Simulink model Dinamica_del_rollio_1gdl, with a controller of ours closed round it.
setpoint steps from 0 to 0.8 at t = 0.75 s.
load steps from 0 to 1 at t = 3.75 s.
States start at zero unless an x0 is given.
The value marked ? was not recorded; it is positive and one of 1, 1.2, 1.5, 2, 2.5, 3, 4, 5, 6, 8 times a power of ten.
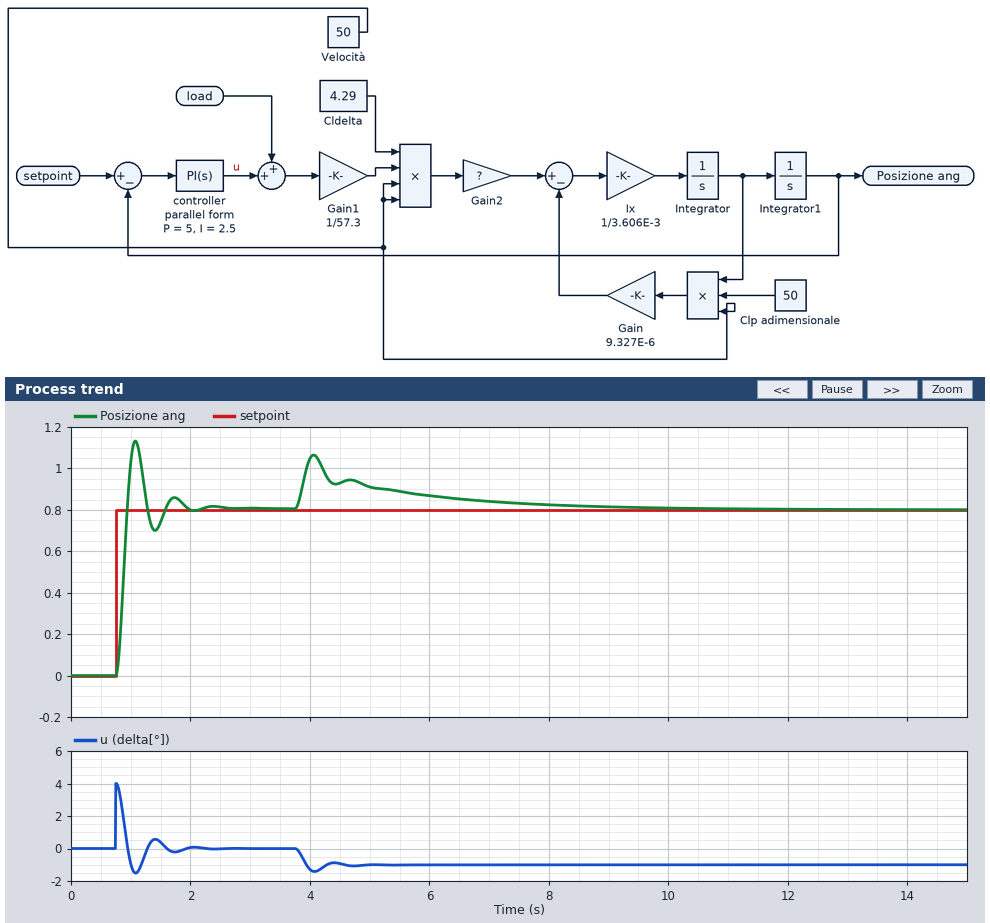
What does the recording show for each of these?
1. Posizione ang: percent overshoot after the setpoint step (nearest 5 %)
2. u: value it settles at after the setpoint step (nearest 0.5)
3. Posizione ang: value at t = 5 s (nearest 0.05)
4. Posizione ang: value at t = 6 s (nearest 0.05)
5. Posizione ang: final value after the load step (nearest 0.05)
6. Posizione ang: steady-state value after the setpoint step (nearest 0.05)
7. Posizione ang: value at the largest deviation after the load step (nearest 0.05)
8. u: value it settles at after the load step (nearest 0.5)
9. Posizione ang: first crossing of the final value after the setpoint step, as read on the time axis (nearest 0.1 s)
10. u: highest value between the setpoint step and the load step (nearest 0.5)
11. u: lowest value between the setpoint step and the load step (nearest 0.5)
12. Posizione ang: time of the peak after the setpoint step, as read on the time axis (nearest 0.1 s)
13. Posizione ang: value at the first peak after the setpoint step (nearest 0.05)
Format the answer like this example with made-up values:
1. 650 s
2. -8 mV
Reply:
1. 40 %
2. 0.0
3. 0.90
4. 0.85
5. 0.80
6. 0.80
7. 1.05
8. -1.0
9. 0.9 s
10. 4.0
11. -1.5
12. 1.1 s
13. 1.15
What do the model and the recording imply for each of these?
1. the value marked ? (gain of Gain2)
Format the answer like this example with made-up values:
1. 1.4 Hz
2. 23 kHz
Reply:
1. 0.0004
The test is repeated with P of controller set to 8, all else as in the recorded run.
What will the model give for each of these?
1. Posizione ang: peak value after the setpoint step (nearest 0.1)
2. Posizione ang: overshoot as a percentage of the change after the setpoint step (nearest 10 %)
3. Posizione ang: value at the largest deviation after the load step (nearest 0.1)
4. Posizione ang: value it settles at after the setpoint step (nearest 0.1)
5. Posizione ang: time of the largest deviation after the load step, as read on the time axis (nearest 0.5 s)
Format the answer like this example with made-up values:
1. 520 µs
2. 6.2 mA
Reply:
1. 1.2
2. 50 %
3. 1.0
4. 0.8
5. 4.0 s
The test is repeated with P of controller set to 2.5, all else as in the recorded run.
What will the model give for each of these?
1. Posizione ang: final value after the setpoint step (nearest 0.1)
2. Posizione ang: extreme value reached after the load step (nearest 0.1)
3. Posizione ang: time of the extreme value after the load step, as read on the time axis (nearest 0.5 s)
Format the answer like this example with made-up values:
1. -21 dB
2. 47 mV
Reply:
1. 0.8
2. 1.2
3. 4.0 s
